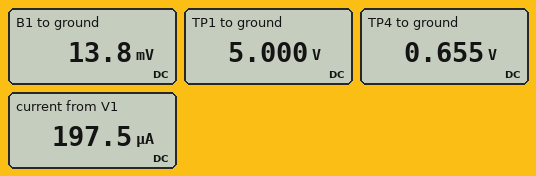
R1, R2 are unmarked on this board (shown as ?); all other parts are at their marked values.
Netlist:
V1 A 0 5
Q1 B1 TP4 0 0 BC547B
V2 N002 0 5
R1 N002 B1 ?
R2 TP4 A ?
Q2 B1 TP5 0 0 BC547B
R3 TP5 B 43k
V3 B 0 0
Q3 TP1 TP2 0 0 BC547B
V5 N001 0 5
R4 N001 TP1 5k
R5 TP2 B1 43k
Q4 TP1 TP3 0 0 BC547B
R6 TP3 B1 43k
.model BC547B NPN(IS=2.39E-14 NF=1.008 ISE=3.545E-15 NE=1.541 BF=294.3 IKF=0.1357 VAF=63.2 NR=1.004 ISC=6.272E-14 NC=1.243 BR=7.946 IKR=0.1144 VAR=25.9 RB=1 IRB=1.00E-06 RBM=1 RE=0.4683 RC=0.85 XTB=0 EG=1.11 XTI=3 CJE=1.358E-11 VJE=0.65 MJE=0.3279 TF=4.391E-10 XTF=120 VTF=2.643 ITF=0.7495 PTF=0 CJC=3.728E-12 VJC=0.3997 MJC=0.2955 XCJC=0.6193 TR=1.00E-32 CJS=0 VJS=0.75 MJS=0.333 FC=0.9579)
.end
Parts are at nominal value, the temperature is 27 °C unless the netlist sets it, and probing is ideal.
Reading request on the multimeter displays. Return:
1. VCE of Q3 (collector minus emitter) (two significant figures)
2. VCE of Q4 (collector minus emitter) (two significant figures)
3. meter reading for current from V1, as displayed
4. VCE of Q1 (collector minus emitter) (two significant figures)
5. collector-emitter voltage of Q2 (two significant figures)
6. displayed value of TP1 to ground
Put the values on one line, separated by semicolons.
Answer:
5.0 V; 5.0 V; 197.5 µA; 14 mV; 14 mV; 5.000 V
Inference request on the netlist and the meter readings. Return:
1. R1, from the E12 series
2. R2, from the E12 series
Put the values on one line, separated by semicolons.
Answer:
12 kΩ; 22 kΩ
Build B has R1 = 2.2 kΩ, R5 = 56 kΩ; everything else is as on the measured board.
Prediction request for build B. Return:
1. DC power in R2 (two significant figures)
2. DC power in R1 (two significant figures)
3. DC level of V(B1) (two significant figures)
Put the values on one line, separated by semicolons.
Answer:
850 µW; 11 mW; 35 mV
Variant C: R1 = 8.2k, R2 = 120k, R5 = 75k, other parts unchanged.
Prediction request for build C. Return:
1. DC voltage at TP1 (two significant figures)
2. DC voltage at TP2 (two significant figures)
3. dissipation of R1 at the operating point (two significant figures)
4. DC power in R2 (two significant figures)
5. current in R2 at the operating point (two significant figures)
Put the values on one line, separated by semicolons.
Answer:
5.0 V; 40 mV; 3.0 mW; 160 µW; 36 µA
